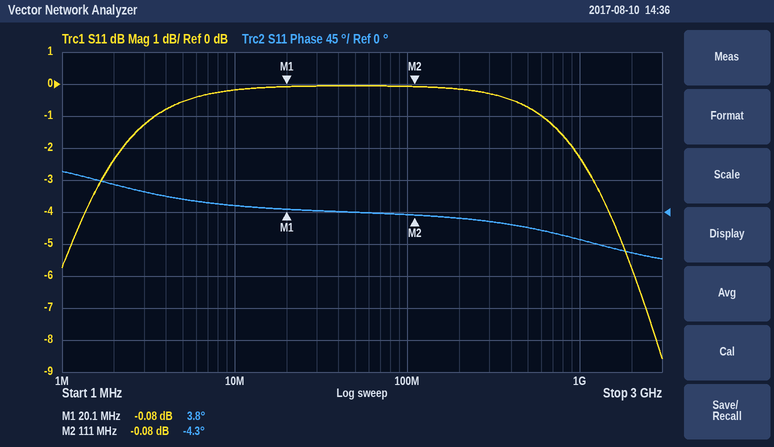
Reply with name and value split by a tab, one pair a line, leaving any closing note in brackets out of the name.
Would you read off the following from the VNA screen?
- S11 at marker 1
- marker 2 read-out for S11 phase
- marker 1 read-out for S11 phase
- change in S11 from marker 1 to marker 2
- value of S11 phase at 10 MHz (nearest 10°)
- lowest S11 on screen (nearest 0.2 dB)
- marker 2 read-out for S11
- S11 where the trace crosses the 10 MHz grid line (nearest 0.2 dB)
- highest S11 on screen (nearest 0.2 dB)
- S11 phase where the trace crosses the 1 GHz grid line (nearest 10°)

S11 at marker 1	-0.08 dB
marker 2 read-out for S11 phase	-4.3°
marker 1 read-out for S11 phase	3.8°
change in S11 from marker 1 to marker 2	0.00 dB
value of S11 phase at 10 MHz	10°
lowest S11 on screen	-8.6 dB
marker 2 read-out for S11	-0.08 dB
S11 where the trace crosses the 10 MHz grid line	-0.2 dB
highest S11 on screen	0.0 dB
S11 phase where the trace crosses the 1 GHz grid line	-40°
